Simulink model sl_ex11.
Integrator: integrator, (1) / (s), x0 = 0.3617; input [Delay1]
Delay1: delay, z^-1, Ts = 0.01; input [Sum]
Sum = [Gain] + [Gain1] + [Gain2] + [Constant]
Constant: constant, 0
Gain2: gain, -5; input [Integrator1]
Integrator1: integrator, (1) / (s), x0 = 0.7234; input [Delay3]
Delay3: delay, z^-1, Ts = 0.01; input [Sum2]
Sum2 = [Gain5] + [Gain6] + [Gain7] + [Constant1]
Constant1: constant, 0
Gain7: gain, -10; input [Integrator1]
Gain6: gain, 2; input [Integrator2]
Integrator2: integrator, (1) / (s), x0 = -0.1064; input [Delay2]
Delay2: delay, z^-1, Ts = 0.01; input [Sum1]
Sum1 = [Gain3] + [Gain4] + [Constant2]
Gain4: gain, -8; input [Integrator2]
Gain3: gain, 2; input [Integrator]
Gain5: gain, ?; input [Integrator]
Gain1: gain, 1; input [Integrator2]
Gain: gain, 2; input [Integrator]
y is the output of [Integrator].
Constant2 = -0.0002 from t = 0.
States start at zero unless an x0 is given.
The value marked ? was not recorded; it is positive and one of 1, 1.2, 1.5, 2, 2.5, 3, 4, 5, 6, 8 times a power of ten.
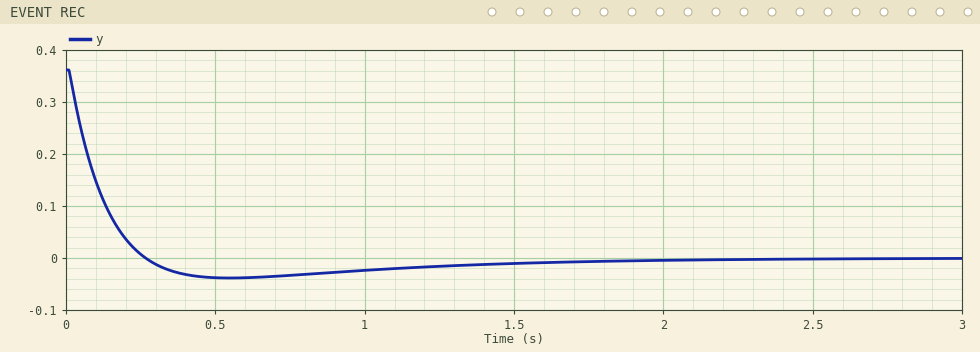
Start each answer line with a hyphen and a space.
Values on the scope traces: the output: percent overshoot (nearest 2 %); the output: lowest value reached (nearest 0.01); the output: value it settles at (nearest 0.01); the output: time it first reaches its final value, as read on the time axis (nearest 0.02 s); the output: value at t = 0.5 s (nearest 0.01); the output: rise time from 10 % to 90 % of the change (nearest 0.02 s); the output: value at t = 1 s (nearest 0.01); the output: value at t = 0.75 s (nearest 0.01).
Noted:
- 10 %
- -0.04
- 0.00
- 0.26 s
- -0.04
- 0.18 s
- -0.02
- -0.03
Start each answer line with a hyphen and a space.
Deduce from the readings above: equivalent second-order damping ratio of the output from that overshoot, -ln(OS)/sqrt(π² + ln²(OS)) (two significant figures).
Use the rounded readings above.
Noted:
- 0.59
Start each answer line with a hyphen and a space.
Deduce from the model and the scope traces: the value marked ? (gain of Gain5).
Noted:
- 6
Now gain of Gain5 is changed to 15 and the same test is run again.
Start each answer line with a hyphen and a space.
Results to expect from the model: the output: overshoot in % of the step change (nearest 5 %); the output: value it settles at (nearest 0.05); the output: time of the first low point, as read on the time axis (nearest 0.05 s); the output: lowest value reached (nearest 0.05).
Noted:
- 35 %
- 0.00
- 0.30 s
- -0.15
